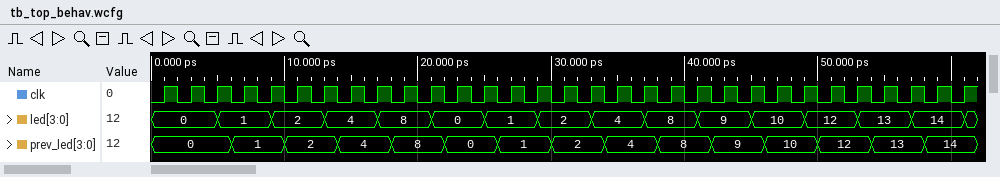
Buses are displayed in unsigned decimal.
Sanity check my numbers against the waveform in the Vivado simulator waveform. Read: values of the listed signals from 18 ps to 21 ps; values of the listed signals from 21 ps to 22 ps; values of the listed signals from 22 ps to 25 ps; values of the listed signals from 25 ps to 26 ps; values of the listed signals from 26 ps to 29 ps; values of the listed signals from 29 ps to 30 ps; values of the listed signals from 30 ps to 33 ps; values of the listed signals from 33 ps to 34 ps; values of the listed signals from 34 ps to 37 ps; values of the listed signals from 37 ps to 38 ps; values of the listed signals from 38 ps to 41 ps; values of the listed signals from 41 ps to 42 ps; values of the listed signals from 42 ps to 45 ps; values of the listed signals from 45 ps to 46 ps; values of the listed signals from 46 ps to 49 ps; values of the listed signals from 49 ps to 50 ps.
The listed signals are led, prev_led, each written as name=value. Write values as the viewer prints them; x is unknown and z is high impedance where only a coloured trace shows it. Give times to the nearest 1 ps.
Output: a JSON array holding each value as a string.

["led=8, prev_led=8", "led=0, prev_led=8", "led=0, prev_led=0", "led=1, prev_led=0", "led=1, prev_led=1", "led=2, prev_led=1", "led=2, prev_led=2", "led=4, prev_led=2", "led=4, prev_led=4", "led=8, prev_led=4", "led=8, prev_led=8", "led=9, prev_led=8", "led=9, prev_led=9", "led=10, prev_led=9", "led=10, prev_led=10", "led=12, prev_led=10"]
